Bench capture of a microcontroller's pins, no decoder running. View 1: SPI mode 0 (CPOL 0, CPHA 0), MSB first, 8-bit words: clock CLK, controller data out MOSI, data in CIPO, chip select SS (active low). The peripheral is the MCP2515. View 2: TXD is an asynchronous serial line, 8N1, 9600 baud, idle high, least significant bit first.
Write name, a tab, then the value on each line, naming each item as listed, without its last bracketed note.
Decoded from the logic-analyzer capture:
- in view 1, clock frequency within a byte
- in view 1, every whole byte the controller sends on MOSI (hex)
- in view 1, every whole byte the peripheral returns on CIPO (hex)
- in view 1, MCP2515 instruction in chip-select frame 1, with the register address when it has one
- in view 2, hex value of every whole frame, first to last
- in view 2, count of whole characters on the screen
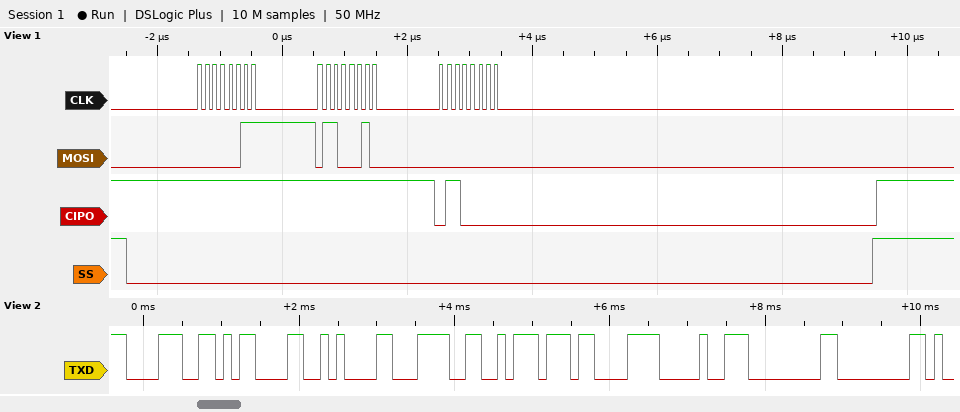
in view 1, clock frequency within a byte	8 MHz
in view 1, every whole byte the controller sends on MOSI	0x03 0x62 0x00
in view 1, every whole byte the peripheral returns on CIPO	0xFF 0xFF 0x60
in view 1, MCP2515 instruction in chip-select frame 1, with the register address when it has one	READ 0x62
in view 2, hex value of every whole frame, first to last	38 0D 0A 3C BA C3 90 00 00
in view 2, count of whole characters on the screen	9
